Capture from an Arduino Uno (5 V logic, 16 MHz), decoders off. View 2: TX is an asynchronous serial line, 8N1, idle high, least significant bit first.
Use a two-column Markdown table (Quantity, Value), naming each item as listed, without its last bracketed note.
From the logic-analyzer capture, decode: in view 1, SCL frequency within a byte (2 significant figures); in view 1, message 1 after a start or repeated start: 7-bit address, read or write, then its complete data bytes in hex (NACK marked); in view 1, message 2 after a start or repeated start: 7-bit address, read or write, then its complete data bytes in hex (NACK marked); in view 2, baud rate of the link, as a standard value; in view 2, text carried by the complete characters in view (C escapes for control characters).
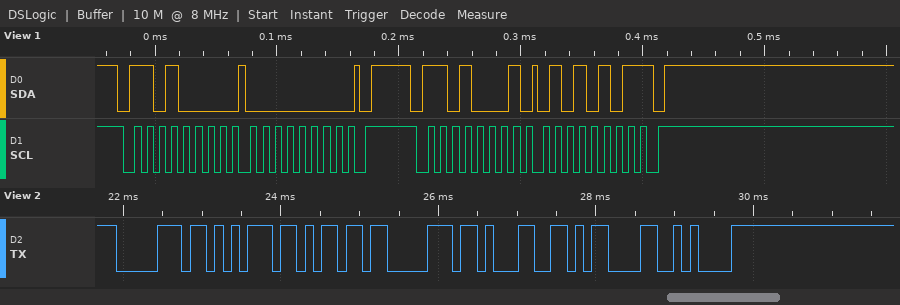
| Quantity | Value |
|---|---|
| in view 1, SCL frequency within a byte | 100 kHz |
| in view 1, message 1 after a start or repeated start: 7-bit address, read or write, then its complete data bytes in hex | 0x68 write: 00 |
| in view 1, message 2 after a start or repeated start: 7-bit address, read or write, then its complete data bytes in hex | 0x68 read: 55 NACK |
| in view 2, baud rate of the link, as a standard value | 9600 baud |
| in view 2, text carried by the complete characters in view | "pump1\r\n" |
